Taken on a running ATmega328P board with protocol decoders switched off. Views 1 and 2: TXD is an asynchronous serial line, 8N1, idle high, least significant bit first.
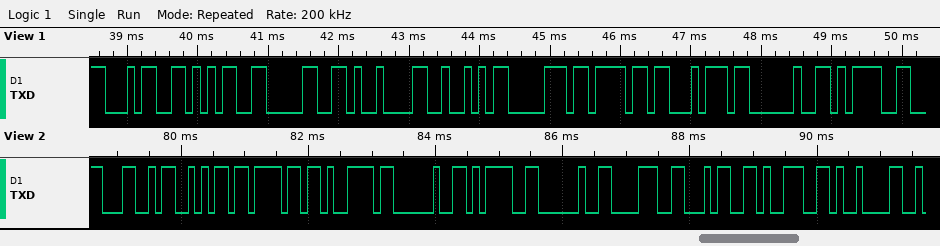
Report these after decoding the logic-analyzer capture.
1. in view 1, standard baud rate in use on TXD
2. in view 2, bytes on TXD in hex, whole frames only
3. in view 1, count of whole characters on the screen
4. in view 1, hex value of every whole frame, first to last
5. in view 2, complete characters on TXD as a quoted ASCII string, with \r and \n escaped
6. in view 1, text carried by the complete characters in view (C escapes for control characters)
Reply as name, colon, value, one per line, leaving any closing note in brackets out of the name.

in view 1, standard baud rate in use on TXD: 9600 baud
in view 2, bytes on TXD in hex, whole frames only: 4C 6A 6F 79 20 3D 20 38 34 39 09
in view 1, count of whole characters on the screen: 10
in view 1, hex value of every whole frame, first to last: 34 35 30 09 52 70 6F 74 20 3D
in view 2, complete characters on TXD as a quoted ASCII string, with \r and \n escaped: "Ljoy = 849\t"
in view 1, text carried by the complete characters in view: "450\tRpot ="
